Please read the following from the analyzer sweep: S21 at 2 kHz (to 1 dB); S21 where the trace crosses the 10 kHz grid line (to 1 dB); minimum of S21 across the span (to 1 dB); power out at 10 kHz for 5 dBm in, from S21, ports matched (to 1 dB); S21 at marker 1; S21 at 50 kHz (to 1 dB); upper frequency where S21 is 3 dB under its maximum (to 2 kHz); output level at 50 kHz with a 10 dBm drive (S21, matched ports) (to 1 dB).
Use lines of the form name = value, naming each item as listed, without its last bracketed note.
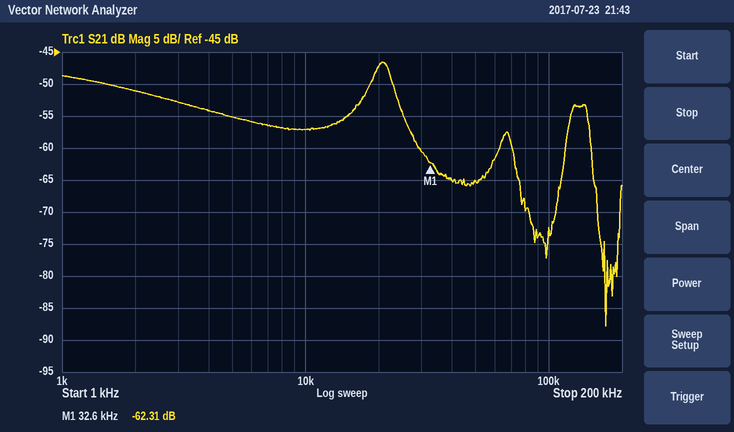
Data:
S21 at 2 kHz = -51 dB
S21 where the trace crosses the 10 kHz grid line = -57 dB
minimum of S21 across the span = -88 dB
power out at 10 kHz for 5 dBm in, from S21, ports matched = -52 dBm
S21 at marker 1 = -62.31 dB
S21 at 50 kHz = -65 dB
upper frequency where S21 is 3 dB under its maximum = 22 kHz
output level at 50 kHz with a 10 dBm drive (S21, matched ports) = -55 dBm
